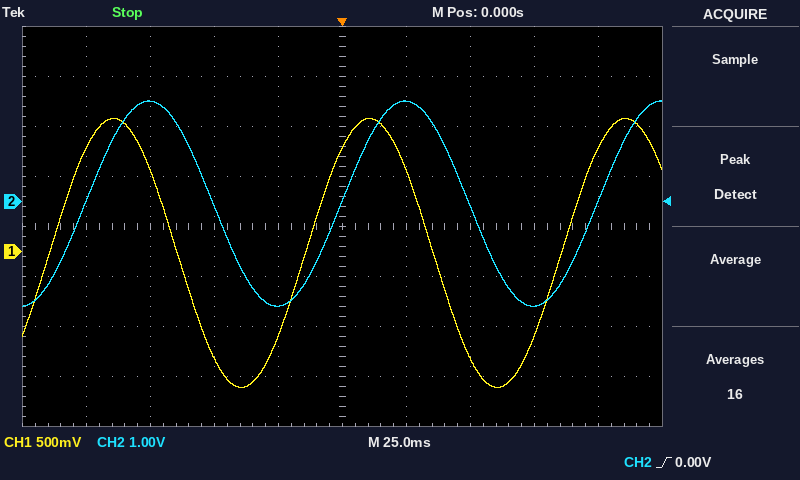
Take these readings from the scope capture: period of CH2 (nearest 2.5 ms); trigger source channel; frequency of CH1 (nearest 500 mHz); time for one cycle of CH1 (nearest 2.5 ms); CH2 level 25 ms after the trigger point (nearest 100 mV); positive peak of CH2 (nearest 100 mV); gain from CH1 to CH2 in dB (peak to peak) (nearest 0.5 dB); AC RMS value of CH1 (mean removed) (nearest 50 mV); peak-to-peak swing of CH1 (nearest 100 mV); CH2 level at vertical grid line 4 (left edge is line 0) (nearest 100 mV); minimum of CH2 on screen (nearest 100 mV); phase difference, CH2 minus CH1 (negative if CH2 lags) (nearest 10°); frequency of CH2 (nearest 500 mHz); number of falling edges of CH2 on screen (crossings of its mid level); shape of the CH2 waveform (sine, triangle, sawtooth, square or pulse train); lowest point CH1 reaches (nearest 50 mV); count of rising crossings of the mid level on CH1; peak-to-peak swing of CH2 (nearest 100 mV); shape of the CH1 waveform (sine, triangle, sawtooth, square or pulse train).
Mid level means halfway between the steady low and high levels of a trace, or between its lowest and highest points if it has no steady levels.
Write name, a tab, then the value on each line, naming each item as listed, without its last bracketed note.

period of CH2	100.0 ms
trigger source channel	CH2
frequency of CH1	10.0 Hz
time for one cycle of CH1	100.0 ms
CH2 level 25 ms after the trigger point	2.0 V
positive peak of CH2	2.0 V
gain from CH1 to CH2 in dB (peak to peak)	3.5 dB
AC RMS value of CH1 (mean removed)	950 mV
peak-to-peak swing of CH1	2.70 V
CH2 level at vertical grid line 4 (left edge is line 0)	-2.1 V
minimum of CH2 on screen	-2.1 V
phase difference, CH2 minus CH1 (negative if CH2 lags)	-50°
frequency of CH2	10.0 Hz
number of falling edges of CH2 on screen	2
shape of the CH2 waveform	sine
lowest point CH1 reaches	-1.35 V
count of rising crossings of the mid level on CH1	3
peak-to-peak swing of CH2	4.1 V
shape of the CH1 waveform	sine
